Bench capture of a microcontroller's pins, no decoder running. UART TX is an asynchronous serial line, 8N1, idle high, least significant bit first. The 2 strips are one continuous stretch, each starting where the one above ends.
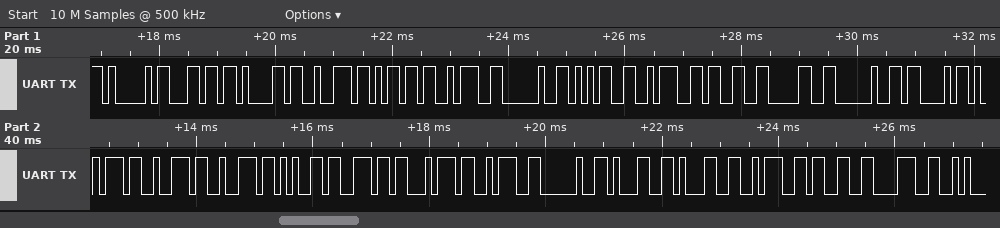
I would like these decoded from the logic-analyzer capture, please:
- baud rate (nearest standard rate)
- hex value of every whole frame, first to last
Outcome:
9600 baud
41 6C 61 72 6D 3A 20 35 3A 33 30 20 43 75 72 72 65 6E 74 3A 20 31 31 3A 33 38
